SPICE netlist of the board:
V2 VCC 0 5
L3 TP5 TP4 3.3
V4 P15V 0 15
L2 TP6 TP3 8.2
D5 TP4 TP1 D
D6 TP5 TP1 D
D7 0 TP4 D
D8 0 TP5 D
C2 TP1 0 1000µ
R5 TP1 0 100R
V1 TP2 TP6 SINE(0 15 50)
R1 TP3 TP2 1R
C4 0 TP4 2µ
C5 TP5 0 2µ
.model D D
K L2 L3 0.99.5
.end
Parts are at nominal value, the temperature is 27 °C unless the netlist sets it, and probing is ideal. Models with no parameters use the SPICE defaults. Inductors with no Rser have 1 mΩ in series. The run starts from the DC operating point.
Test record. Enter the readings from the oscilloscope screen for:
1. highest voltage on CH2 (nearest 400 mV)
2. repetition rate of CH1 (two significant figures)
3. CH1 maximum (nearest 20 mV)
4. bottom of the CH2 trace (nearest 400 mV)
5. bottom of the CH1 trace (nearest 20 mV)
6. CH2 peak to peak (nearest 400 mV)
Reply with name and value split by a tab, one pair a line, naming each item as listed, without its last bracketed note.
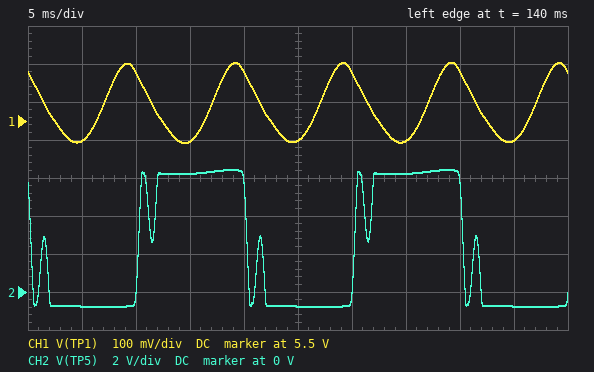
highest voltage on CH2	6.4 V
repetition rate of CH1	100 Hz
CH1 maximum	5.66 V
bottom of the CH2 trace	-800 mV
bottom of the CH1 trace	5.44 V
CH2 peak to peak	7.2 V
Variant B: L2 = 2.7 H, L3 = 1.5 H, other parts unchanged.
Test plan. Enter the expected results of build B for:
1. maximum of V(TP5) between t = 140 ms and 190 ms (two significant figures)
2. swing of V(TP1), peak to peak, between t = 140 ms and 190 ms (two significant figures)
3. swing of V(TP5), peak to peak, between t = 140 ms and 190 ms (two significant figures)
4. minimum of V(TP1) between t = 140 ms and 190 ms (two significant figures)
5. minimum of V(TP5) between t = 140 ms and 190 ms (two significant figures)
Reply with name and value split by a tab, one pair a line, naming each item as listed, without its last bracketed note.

maximum of V(TP5) between t = 140 ms and 190 ms	8.4 V
swing of V(TP1), peak to peak, between t = 140 ms and 190 ms	360 mV
swing of V(TP5), peak to peak, between t = 140 ms and 190 ms	9.2 V
minimum of V(TP1) between t = 140 ms and 190 ms	7.3 V
minimum of V(TP5) between t = 140 ms and 190 ms	-790 mV
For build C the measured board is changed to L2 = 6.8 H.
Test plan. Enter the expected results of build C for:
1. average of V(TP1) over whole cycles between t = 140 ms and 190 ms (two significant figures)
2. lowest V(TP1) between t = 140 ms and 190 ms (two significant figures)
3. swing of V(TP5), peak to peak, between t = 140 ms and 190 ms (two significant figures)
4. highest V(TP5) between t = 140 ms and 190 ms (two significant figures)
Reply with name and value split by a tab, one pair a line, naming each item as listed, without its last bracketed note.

average of V(TP1) over whole cycles between t = 140 ms and 190 ms	6.2 V
lowest V(TP1) between t = 140 ms and 190 ms	6.1 V
swing of V(TP5), peak to peak, between t = 140 ms and 190 ms	7.9 V
highest V(TP5) between t = 140 ms and 190 ms	7.1 V
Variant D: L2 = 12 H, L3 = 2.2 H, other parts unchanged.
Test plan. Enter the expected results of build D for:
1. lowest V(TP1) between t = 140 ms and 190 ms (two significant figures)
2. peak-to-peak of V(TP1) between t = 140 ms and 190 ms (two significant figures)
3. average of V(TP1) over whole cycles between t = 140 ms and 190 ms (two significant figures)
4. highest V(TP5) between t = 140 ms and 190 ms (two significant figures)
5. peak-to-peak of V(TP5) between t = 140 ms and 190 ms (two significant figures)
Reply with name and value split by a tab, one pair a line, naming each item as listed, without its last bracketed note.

lowest V(TP1) between t = 140 ms and 190 ms	3.5 V
peak-to-peak of V(TP1) between t = 140 ms and 190 ms	160 mV
average of V(TP1) over whole cycles between t = 140 ms and 190 ms	3.6 V
highest V(TP5) between t = 140 ms and 190 ms	4.4 V
peak-to-peak of V(TP5) between t = 140 ms and 190 ms	5.2 V
